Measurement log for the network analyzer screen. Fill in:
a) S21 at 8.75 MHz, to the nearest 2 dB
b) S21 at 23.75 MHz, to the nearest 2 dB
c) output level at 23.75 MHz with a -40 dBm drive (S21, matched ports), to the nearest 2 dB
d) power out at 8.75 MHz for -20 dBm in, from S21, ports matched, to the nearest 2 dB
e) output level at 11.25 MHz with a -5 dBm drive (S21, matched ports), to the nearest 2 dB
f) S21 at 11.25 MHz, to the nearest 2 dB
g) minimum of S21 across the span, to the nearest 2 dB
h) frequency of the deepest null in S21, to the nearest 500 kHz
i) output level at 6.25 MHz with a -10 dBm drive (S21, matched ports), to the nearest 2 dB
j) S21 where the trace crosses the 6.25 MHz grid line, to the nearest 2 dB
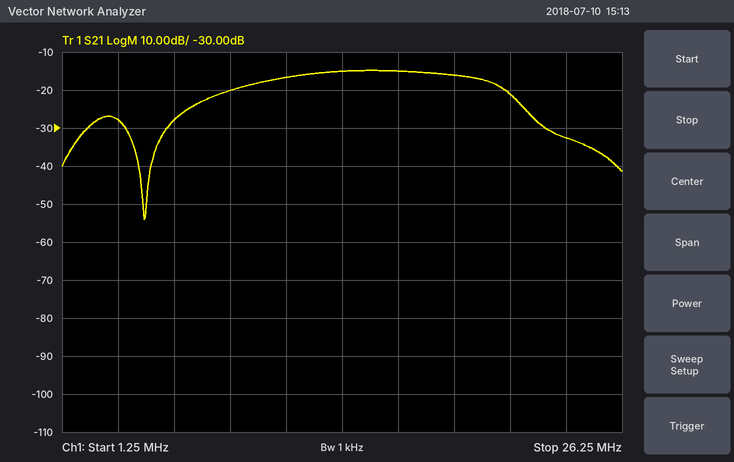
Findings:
-20 dB
-32 dB
-72 dBm
-40 dBm
-22 dBm
-16 dB
-54 dB
5.0 MHz
-38 dBm
-28 dB
